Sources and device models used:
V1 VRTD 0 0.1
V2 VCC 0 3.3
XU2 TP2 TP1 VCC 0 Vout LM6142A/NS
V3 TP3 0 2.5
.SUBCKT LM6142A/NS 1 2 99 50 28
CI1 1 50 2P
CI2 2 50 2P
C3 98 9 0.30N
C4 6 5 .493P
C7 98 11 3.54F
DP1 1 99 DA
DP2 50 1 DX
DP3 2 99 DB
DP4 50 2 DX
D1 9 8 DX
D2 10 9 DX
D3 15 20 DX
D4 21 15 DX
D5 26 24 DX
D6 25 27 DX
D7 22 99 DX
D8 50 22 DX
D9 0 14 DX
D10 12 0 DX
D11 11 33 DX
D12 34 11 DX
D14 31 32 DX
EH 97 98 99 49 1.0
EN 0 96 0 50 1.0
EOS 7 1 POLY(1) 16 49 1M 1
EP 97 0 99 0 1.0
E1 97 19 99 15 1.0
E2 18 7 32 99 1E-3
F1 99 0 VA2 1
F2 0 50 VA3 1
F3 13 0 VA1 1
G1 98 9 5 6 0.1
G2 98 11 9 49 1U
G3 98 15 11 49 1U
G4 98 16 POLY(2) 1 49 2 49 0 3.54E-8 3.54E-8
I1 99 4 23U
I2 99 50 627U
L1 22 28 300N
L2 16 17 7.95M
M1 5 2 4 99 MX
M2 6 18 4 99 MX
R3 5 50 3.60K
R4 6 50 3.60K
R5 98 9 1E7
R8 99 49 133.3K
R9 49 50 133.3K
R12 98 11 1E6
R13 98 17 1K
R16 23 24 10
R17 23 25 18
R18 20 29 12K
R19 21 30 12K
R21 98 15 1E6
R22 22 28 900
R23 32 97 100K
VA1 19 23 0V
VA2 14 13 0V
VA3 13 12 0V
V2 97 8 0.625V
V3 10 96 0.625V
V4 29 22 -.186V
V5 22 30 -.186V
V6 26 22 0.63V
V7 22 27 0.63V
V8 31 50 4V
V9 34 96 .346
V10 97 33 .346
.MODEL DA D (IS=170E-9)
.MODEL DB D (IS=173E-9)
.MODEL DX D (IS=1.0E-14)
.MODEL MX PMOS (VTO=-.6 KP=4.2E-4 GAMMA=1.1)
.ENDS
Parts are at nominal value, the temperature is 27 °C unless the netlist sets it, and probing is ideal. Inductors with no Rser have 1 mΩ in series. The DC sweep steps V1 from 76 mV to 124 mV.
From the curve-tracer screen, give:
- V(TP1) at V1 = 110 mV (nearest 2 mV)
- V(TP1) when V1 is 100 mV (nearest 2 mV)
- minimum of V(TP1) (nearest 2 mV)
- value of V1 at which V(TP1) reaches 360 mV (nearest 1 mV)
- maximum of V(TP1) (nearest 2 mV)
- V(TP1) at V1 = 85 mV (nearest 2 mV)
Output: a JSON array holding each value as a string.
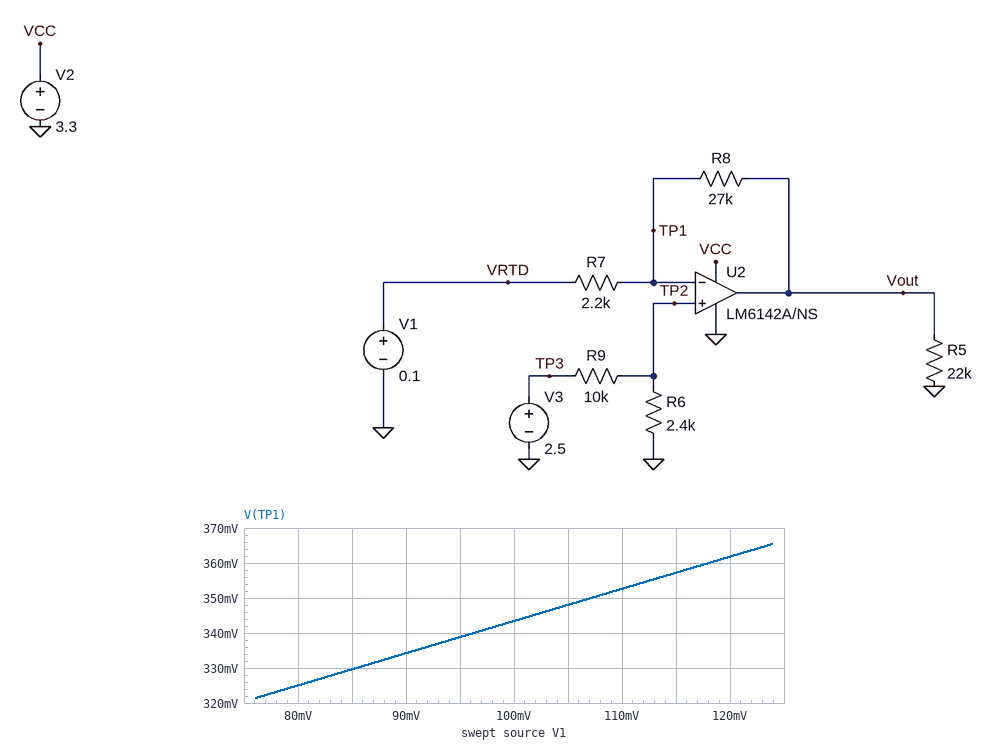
["352 mV", "344 mV", "322 mV", "118 mV", "366 mV", "330 mV"]
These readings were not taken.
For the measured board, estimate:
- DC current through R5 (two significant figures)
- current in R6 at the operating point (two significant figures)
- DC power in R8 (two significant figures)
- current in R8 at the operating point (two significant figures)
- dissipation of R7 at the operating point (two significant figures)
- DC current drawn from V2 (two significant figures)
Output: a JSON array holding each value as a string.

["150 µA", "200 µA", "330 µW", "110 µA", "27 µW", "920 µA"]
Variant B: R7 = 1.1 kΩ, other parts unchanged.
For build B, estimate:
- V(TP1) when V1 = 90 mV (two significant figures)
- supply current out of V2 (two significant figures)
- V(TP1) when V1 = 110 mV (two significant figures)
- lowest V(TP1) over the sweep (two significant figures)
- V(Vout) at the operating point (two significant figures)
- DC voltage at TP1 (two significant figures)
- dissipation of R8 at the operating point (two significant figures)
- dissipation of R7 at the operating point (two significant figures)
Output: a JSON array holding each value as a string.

["220 mV", "930 µA", "240 mV", "200 mV", "3.3 V", "230 mV", "360 µW", "15 µW"]
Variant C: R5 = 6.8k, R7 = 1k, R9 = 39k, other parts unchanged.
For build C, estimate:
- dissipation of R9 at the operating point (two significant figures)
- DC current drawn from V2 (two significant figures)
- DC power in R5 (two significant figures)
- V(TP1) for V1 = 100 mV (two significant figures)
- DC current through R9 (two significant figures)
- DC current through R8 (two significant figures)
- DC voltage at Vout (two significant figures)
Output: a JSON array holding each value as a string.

["140 µW", "910 µA", "290 µW", "150 mV", "60 µA", "46 µA", "1.4 V"]
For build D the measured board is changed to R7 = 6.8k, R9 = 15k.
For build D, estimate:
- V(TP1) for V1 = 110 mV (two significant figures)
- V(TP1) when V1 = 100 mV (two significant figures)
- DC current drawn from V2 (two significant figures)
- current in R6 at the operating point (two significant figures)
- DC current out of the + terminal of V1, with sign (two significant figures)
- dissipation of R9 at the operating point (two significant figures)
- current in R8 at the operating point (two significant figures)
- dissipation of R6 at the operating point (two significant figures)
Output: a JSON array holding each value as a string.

["350 mV", "350 mV", "760 µA", "140 µA", "-36 µA", "310 µW", "36 µA", "50 µW"]
